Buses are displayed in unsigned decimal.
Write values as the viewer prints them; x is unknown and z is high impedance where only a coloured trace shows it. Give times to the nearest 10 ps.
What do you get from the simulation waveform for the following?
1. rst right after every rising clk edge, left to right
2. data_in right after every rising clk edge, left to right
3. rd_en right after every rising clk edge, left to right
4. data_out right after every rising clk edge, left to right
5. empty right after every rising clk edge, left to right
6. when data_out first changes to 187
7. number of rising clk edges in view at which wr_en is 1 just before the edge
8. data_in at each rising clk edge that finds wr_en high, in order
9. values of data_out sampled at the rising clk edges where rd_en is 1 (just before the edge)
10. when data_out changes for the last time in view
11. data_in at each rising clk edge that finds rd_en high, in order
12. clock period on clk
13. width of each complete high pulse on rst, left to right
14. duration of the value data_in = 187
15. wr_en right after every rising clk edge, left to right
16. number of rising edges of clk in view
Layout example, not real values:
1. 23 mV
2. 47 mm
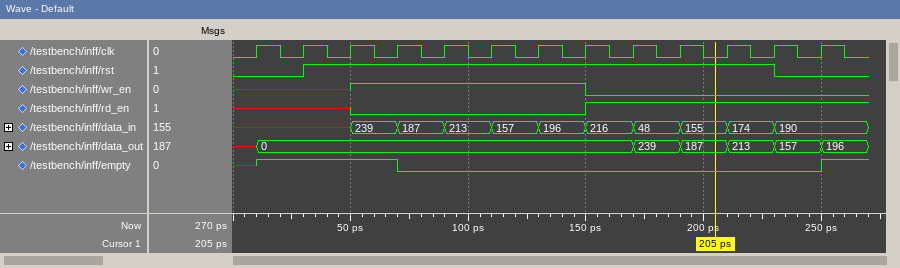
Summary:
1. 0 1 1 1 1 1 1 1 1 1 1 0 0
2. x, x, 239, 187, 213, 157, 196, 216, 48, 155, 174, 190, 190
3. x x 0 0 0 0 0 1 1 1 1 1 1
4. 0, 0, 0, 0, 0, 0, 0, 0, 239, 187, 213, 157, 196
5. 1 1 1 0 0 0 0 0 0 0 0 0 1
6. 190 ps
7. 5
8. 239, 187, 213, 157, 196
9. 0, 239, 187, 213, 157
10. 250 ps
11. 216, 48, 155, 174, 190
12. 20 ps
13. 200 ps
14. 20 ps
15. x x 1 1 1 1 1 0 0 0 0 0 0
16. 13
